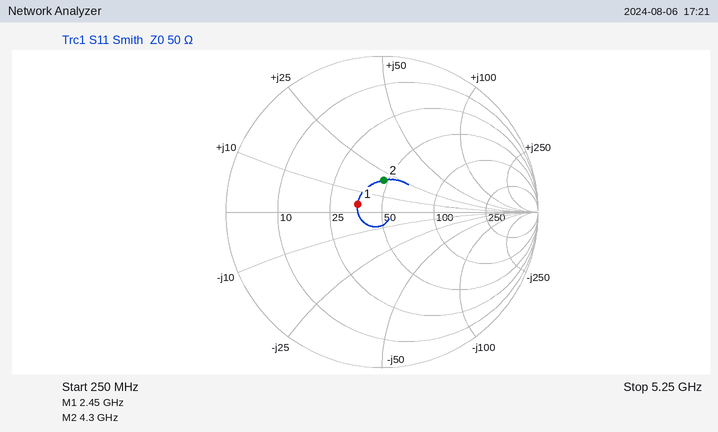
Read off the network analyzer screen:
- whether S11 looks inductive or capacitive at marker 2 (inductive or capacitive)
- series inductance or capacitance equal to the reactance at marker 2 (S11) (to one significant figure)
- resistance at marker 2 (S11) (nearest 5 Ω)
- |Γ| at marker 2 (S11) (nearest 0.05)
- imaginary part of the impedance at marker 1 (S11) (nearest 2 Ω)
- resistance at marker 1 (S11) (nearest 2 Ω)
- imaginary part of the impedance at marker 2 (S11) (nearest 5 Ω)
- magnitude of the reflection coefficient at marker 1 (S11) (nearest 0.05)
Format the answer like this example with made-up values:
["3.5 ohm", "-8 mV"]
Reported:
["inductive", "700 pH", "45 Ω", "0.20", "+4 Ω", "36 Ω", "+20 Ω", "0.15"]
